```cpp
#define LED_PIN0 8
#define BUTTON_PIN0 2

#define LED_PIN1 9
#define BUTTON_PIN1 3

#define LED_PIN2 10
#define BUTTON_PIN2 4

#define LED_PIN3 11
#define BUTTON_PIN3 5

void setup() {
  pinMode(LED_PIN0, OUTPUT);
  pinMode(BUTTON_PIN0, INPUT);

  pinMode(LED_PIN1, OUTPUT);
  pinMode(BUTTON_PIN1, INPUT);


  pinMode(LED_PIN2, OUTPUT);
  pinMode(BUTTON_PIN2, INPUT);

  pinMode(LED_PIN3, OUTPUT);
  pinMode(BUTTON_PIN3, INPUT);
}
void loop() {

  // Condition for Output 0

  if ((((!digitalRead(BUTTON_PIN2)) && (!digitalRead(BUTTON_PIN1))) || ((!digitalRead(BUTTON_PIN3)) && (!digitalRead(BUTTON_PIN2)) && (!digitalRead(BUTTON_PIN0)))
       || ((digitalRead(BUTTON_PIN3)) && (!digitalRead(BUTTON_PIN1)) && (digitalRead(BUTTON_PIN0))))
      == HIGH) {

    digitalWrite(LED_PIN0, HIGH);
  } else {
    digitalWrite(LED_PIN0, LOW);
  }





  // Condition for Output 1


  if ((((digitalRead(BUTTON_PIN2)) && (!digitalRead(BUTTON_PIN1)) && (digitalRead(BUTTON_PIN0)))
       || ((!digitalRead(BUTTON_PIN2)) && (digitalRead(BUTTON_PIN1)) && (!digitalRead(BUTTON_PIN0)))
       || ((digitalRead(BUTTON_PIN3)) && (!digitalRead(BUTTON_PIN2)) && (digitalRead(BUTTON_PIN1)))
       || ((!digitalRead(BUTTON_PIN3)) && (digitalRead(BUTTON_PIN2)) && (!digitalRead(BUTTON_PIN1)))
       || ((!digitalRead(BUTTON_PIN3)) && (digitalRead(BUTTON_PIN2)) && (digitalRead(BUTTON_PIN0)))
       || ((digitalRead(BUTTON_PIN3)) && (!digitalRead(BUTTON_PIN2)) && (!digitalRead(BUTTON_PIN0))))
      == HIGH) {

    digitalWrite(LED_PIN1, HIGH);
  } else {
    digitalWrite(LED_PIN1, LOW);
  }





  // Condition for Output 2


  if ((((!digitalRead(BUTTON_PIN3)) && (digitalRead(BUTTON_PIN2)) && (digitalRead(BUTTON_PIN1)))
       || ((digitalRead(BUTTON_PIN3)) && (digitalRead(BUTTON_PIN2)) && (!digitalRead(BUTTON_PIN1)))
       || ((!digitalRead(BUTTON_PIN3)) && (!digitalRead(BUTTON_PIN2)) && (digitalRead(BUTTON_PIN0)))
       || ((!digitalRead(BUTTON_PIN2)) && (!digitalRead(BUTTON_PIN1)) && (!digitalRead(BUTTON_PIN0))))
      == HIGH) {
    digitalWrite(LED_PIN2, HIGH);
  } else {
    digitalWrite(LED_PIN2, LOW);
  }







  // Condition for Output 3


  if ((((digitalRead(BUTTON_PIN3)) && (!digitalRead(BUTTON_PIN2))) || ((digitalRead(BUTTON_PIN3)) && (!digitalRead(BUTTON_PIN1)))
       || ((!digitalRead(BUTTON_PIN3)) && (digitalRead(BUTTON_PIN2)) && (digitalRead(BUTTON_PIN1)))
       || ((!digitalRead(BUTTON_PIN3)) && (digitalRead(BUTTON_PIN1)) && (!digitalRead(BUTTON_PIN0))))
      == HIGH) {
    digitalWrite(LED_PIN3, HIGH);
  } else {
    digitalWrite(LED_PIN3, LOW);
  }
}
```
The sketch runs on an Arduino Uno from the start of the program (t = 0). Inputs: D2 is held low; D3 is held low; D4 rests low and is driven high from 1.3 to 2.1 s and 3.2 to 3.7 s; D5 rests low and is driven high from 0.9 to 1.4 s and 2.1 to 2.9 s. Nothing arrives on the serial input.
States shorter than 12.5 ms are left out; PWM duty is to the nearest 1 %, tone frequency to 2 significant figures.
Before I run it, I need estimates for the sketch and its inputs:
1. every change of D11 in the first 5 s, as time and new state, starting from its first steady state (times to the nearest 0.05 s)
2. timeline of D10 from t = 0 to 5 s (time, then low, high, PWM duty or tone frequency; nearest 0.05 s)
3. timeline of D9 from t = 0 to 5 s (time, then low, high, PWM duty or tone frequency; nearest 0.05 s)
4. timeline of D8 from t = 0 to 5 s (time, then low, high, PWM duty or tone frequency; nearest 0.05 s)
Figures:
0 s low; 0.9 s high; 1.4 s low; 2.1 s high; 2.9 s low
0 s high; 1.4 s low; 2.1 s high; 3.2 s low; 3.7 s high
0 s low; 0.9 s high; 1.3 s low; 1.4 s high; 2.9 s low; 3.2 s high; 3.7 s low
0 s high; 1.3 s low; 2.1 s high; 3.2 s low; 3.7 s high
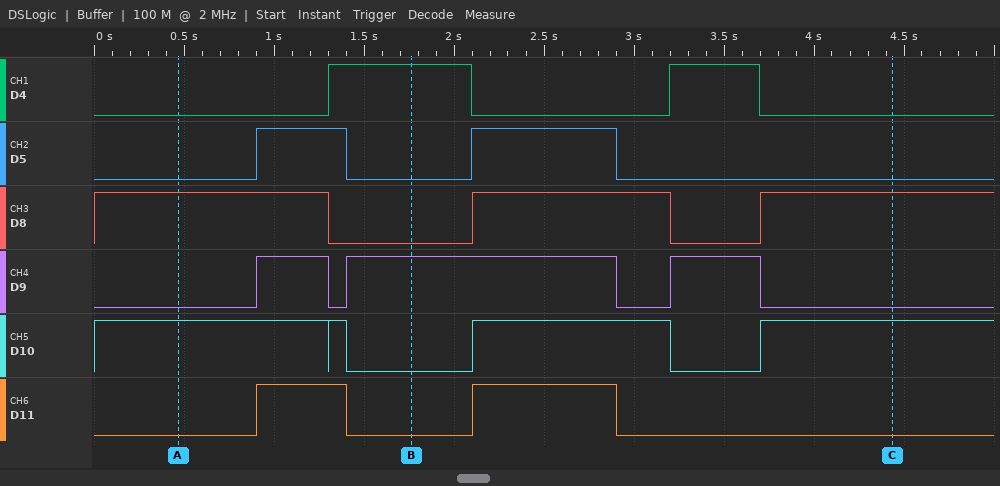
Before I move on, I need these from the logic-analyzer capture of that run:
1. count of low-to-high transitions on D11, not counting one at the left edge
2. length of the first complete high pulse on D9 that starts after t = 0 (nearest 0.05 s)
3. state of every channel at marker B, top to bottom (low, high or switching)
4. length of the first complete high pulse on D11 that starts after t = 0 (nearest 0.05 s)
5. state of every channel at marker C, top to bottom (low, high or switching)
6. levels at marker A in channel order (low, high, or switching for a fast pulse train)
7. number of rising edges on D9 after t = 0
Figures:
2
0.40 s
D4 high, D5 low, D8 low, D9 high, D10 low, D11 low
0.50 s
D4 low, D5 low, D8 high, D9 low, D10 high, D11 low
D4 low, D5 low, D8 high, D9 low, D10 high, D11 low
3
